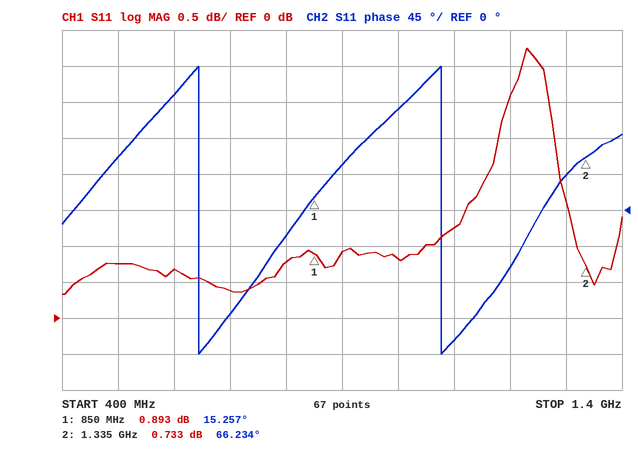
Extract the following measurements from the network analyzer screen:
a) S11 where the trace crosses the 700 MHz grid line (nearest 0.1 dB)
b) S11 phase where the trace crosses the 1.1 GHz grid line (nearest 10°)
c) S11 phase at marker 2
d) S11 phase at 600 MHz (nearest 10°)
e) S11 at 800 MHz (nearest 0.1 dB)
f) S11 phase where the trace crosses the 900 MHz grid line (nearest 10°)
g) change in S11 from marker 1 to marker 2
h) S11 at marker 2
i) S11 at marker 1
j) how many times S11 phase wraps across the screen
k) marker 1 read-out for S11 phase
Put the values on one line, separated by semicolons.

0.4 dB; -160°; 66.234°; 140°; 0.8 dB; 60°; -0.160 dB; 0.733 dB; 0.893 dB; 2; 15.257°
